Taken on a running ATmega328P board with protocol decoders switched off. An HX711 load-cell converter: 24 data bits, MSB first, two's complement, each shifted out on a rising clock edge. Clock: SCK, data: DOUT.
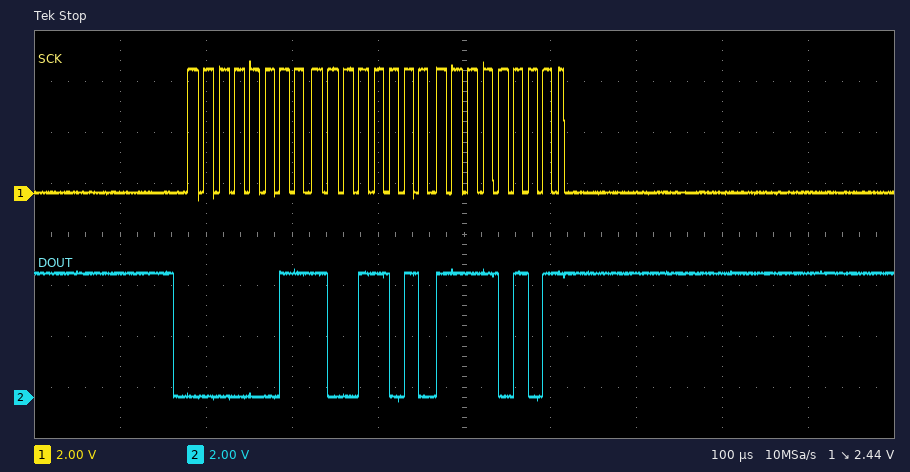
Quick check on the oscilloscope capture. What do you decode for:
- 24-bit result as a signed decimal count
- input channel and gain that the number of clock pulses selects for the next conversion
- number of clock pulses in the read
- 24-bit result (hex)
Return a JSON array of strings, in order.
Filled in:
["236277", "channel A, gain 128", "25", "0x039AF5"]
